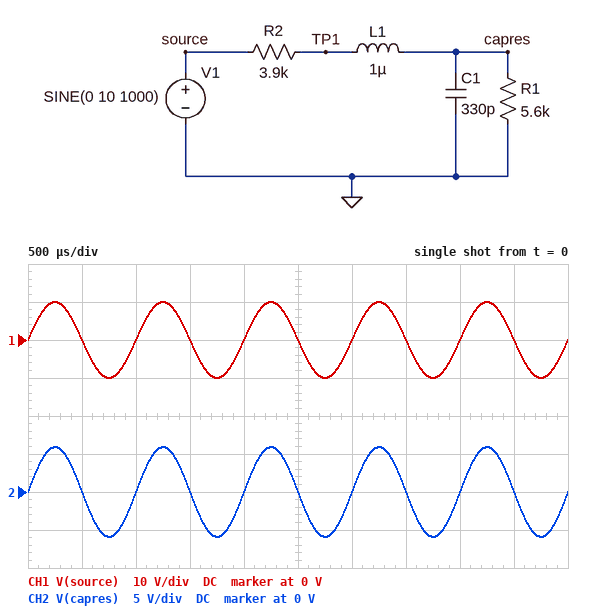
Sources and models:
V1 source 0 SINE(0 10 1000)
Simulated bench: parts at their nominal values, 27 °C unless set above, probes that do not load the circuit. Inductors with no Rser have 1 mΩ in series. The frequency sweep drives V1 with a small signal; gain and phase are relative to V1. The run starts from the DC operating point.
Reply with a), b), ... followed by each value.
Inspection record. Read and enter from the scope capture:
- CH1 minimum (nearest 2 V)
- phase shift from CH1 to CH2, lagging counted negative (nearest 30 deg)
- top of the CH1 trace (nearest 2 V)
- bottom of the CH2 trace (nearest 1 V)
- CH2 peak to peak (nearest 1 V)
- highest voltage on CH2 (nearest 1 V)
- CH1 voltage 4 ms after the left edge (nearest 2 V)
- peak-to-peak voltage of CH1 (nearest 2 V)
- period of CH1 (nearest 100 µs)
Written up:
a) -10 V
b) 0 deg
c) 10 V
d) -6 V
e) 12 V
f) 6 V
g) 0 V
h) 20 V
i) 1.0 ms
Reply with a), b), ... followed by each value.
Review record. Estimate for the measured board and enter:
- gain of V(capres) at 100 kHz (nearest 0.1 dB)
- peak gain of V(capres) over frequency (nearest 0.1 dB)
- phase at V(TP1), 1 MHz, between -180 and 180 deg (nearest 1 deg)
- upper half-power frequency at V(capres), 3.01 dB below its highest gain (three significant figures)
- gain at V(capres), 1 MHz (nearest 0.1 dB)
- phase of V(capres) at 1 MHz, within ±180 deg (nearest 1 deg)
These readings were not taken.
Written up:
a) -5.5 dB
b) -4.6 dB
c) -78 deg
d) 210 kHz
e) -18.3 dB
f) -78 deg
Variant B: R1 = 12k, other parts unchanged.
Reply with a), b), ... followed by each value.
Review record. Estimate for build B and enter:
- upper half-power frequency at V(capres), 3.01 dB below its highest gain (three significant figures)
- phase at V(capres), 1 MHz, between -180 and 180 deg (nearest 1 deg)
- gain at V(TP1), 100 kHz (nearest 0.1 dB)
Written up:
a) 164 kHz
b) -81 deg
c) -3.8 dB
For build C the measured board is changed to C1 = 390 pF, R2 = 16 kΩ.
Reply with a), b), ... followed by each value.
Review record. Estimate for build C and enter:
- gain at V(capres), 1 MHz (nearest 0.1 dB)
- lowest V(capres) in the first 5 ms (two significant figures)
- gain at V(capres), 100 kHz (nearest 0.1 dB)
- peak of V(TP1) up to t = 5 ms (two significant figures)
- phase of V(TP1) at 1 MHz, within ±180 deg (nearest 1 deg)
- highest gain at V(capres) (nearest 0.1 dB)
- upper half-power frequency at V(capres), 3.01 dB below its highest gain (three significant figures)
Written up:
a) -31.9 dB
b) -2.6 V
c) -14.8 dB
d) 2.6 V
e) -84 deg
f) -11.7 dB
g) 98.4 kHz
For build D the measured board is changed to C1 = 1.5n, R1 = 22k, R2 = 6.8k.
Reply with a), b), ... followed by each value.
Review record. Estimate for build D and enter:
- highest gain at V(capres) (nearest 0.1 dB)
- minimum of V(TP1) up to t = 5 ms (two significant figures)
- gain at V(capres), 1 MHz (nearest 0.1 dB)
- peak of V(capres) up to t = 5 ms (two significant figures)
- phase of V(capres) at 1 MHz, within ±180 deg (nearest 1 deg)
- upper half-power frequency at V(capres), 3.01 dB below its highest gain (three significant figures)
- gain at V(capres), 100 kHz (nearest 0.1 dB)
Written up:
a) -2.3 dB
b) -7.6 V
c) -36.1 dB
d) 7.6 V
e) -89 deg
f) 20.4 kHz
g) -16.3 dB
